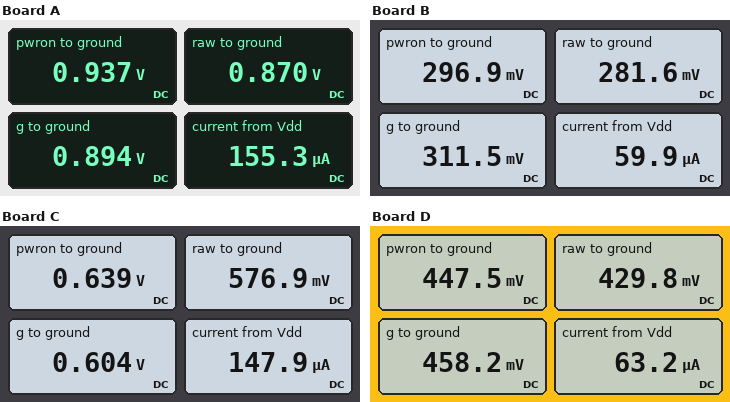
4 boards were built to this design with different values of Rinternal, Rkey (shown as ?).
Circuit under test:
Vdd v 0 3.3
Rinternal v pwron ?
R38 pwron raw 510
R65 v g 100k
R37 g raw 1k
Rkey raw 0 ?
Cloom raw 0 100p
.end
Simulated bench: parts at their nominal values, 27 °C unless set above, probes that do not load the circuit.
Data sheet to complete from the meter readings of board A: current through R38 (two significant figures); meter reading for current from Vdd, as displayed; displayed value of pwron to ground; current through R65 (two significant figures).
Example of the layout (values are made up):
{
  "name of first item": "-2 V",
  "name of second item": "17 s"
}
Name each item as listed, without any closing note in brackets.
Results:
{
  "current through R38": "130 µA",
  "meter reading for current from Vdd, as displayed": "155.3 µA",
  "displayed value of pwron to ground": "0.937 V",
  "current through R65": "24 µA"
}
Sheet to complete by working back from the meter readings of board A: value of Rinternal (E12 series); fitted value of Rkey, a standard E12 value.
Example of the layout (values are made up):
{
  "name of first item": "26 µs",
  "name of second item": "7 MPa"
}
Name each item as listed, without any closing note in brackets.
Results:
{
  "value of Rinternal": "18 kΩ",
  "fitted value of Rkey, a standard E12 value": "5.6 kΩ"
}
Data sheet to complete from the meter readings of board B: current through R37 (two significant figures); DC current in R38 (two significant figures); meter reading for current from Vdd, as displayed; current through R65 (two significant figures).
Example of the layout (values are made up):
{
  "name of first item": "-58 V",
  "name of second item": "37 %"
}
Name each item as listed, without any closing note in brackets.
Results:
{
  "current through R37": "30 µA",
  "DC current in R38": "30 µA",
  "meter reading for current from Vdd, as displayed": "59.9 µA",
  "current through R65": "30 µA"
}
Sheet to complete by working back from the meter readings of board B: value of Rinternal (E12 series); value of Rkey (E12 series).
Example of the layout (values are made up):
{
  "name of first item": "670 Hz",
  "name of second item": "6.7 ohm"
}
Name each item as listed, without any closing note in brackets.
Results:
{
  "value of Rinternal": "100 kΩ",
  "value of Rkey": "4.7 kΩ"
}
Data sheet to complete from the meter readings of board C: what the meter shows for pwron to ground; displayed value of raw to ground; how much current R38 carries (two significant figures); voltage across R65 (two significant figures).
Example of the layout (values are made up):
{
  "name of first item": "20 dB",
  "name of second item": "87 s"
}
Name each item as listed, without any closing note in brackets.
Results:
{
  "what the meter shows for pwron to ground": "0.639 V",
  "displayed value of raw to ground": "576.9 mV",
  "how much current R38 carries": "120 µA",
  "voltage across R65": "2.7 V"
}
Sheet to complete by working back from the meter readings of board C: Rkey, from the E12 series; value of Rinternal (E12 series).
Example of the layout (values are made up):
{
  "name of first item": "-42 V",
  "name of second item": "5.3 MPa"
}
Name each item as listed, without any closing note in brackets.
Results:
{
  "Rkey, from the E12 series": "3.9 kΩ",
  "value of Rinternal": "22 kΩ"
}
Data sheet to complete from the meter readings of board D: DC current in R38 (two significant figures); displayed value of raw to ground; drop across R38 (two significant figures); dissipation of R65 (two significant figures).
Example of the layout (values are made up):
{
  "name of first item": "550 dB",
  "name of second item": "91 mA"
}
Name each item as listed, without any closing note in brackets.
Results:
{
  "DC current in R38": "35 µA",
  "displayed value of raw to ground": "429.8 mV",
  "drop across R38": "18 mV",
  "dissipation of R65": "81 µW"
}
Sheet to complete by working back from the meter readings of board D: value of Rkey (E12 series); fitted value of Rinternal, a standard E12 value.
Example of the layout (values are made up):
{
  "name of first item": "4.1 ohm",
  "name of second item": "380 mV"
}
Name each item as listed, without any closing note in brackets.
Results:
{
  "value of Rkey": "6.8 kΩ",
  "fitted value of Rinternal, a standard E12 value": "82 kΩ"
}
